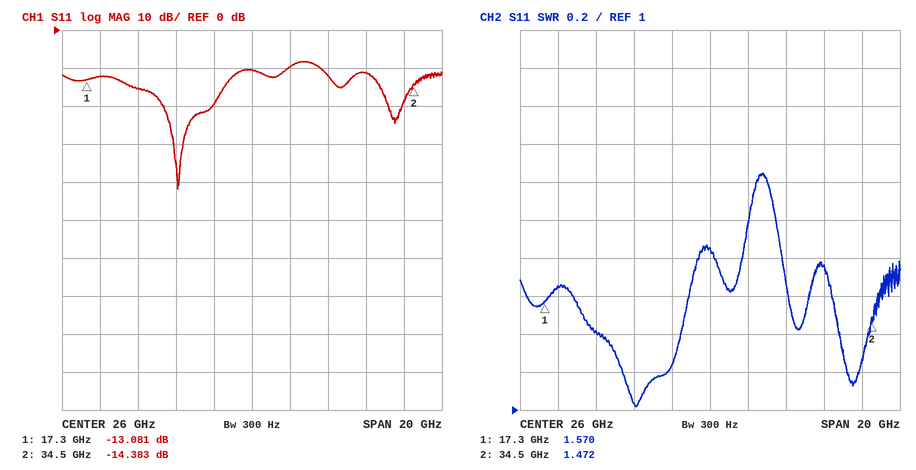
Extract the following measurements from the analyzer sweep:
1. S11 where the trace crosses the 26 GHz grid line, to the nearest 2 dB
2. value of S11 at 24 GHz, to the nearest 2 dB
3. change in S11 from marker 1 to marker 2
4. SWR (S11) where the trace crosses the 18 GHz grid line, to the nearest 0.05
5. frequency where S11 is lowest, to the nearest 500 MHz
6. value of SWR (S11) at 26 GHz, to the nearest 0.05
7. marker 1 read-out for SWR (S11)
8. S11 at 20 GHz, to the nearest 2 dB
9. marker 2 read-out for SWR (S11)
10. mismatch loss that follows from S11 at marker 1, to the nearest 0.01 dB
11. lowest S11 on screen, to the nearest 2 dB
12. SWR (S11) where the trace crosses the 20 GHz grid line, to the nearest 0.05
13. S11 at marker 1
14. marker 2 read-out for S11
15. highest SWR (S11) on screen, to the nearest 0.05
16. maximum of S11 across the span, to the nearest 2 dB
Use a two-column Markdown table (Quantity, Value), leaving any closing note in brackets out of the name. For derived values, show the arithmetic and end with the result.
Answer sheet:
| Quantity | Value |
|---|---|
| S11 where the trace crosses the 26 GHz grid line, to the nearest 2 dB | -10 dB |
| value of S11 at 24 GHz, to the nearest 2 dB | -20 dB |
| change in S11 from marker 1 to marker 2 | -14.383 − (-13.081) = -1.302 dB |
| SWR (S11) where the trace crosses the 18 GHz grid line, to the nearest 0.05 | 1.65 |
| frequency where S11 is lowest, to the nearest 500 MHz | 22.0 GHz |
| value of SWR (S11) at 26 GHz, to the nearest 0.05 | 1.85 |
| marker 1 read-out for SWR | 1.570 |
| S11 at 20 GHz, to the nearest 2 dB | -16 dB |
| marker 2 read-out for SWR | 1.472 |
| mismatch loss that follows from S11 at marker 1, to the nearest 0.01 dB | −10 log10(1 − 10^(-13.081/10)) ≈ 0.22 dB |
| lowest S11 on screen, to the nearest 2 dB | -42 dB |
| SWR (S11) where the trace crosses the 20 GHz grid line, to the nearest 0.05 | 1.40 |
| S11 at marker 1 | -13.081 dB |
| marker 2 read-out for S11 | -14.383 dB |
| highest SWR (S11) on screen, to the nearest 0.05 | 2.25 |
| maximum of S11 across the span, to the nearest 2 dB | -8 dB |
